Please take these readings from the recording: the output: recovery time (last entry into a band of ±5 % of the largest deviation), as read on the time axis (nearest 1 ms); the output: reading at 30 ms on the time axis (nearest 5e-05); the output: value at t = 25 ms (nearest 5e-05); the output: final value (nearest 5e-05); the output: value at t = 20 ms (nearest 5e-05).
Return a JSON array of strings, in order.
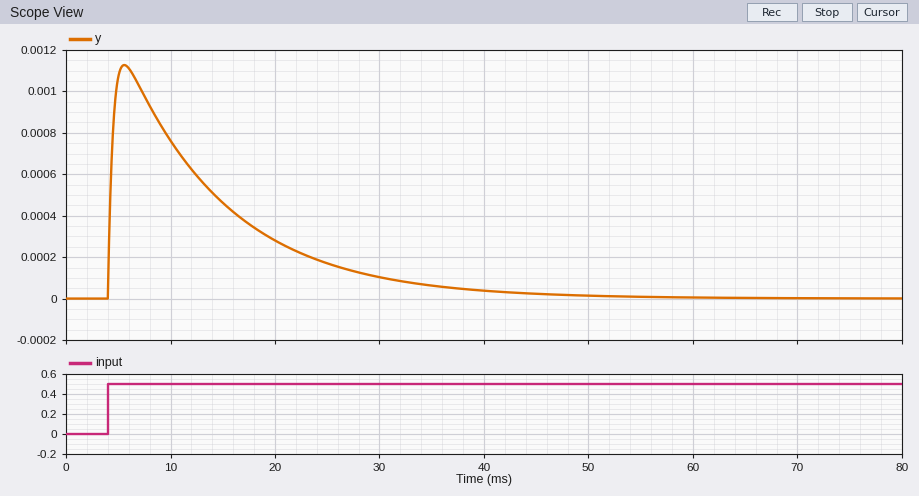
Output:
["36 ms", "0.00010", "0.00015", "0.00000", "0.00030"]
